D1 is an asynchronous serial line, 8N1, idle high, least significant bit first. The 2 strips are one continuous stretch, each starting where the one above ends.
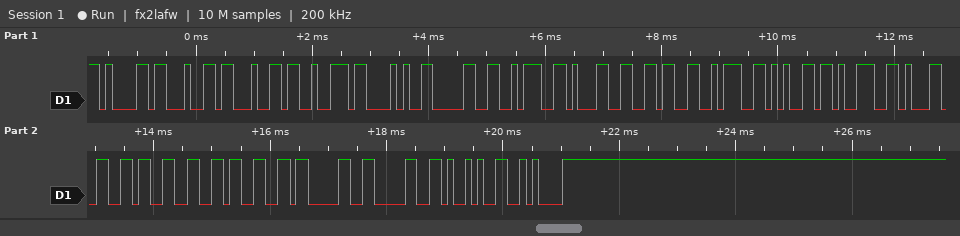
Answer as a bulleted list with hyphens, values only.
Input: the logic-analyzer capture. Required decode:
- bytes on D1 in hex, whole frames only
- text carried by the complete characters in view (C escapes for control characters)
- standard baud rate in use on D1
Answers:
- 61 64 64 72 28 30 3A 31 36 3A 65 39 31 36 66 66 30 30 29 0A
- "addr(0:16:e916ff00)\n"
- 9600 baud
